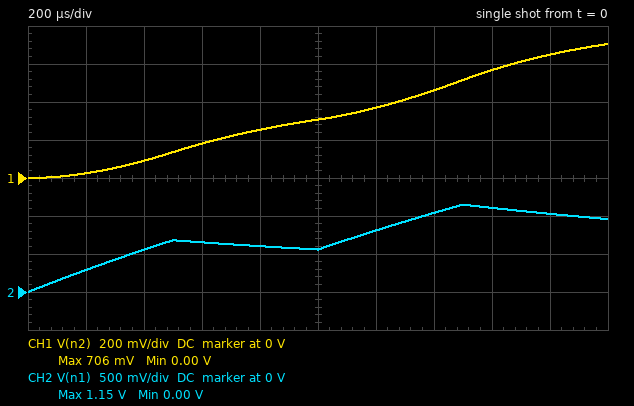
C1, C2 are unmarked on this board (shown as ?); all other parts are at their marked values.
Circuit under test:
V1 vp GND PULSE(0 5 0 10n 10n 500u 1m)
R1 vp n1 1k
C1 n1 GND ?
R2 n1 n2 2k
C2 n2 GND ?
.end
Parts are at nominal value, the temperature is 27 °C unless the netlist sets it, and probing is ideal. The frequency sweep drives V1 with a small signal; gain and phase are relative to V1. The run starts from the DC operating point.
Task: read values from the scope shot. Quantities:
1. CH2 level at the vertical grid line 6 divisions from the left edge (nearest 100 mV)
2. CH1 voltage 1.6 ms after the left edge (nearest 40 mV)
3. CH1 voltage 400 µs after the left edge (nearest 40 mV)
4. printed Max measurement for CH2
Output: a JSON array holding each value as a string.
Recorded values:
["800 mV", "560 mV", "80 mV", "1.15 V"]
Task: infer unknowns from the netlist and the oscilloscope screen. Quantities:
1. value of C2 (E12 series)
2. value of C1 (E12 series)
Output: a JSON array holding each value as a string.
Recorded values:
["560 nF", "3.3 µF"]
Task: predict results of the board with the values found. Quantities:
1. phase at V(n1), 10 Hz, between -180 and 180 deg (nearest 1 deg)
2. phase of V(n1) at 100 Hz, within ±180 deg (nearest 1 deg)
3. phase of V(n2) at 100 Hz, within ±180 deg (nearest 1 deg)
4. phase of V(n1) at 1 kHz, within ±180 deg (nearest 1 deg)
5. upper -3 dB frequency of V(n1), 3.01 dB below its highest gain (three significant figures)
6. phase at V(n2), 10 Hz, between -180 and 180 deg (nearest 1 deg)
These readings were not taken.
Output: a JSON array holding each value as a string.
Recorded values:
["-14 deg", "-63 deg", "-98 deg", "-86 deg", "40.1 Hz", "-18 deg"]
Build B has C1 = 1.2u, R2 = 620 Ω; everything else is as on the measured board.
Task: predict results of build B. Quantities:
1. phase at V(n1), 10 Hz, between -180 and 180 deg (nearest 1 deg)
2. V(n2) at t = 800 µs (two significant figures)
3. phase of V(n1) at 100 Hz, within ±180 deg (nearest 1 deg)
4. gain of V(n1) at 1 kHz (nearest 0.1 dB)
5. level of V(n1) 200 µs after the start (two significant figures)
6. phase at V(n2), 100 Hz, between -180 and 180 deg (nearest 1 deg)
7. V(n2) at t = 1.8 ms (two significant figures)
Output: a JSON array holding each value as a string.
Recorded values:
["-6 deg", "970 mV", "-45 deg", "-18.6 dB", "690 mV", "-58 deg", "1.6 V"]
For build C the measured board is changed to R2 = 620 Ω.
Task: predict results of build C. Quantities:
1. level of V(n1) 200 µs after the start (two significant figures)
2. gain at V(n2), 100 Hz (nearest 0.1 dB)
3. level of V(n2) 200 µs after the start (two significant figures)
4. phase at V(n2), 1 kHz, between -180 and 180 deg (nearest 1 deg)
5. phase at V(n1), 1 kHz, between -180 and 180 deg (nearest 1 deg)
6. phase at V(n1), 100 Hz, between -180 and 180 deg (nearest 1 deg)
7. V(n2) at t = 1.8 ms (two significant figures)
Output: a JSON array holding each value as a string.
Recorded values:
["280 mV", "-8.6 dB", "69 mV", "-149 deg", "-84 deg", "-66 deg", "940 mV"]
